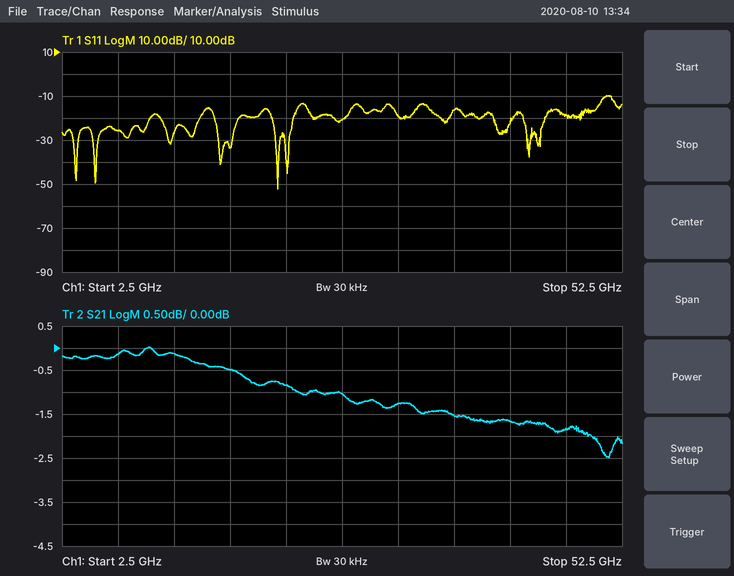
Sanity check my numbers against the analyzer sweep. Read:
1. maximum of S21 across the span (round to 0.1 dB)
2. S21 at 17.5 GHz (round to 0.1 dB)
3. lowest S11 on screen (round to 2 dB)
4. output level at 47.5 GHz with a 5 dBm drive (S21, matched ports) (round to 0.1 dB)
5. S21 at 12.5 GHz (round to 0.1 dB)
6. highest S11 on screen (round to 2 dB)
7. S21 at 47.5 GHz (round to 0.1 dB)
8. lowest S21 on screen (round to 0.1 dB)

0.0 dB
-0.5 dB
-52 dB
3.2 dBm
-0.1 dB
-10 dB
-1.8 dB
-2.5 dB
